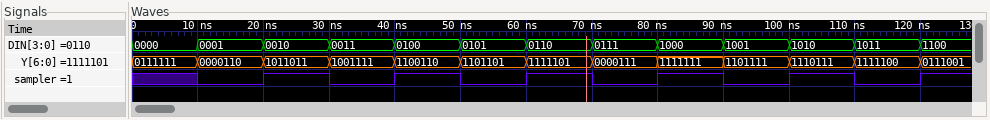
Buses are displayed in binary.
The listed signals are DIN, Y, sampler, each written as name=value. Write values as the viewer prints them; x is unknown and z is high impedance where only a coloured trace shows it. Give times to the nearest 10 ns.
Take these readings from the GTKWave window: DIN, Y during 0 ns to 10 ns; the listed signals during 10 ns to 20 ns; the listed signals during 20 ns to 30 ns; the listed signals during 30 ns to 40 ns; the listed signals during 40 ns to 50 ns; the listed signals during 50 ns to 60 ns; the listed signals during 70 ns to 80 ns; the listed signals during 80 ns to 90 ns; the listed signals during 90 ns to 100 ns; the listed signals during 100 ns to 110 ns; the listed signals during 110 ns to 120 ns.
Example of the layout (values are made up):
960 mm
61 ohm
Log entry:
DIN=0000, Y=0111111
DIN=0001, Y=0000110, sampler=0
DIN=0010, Y=1011011, sampler=1
DIN=0011, Y=1001111, sampler=0
DIN=0100, Y=1100110, sampler=1
DIN=0101, Y=1101101, sampler=0
DIN=0111, Y=0000111, sampler=0
DIN=1000, Y=1111111, sampler=1
DIN=1001, Y=1101111, sampler=0
DIN=1010, Y=1110111, sampler=1
DIN=1011, Y=1111100, sampler=0
